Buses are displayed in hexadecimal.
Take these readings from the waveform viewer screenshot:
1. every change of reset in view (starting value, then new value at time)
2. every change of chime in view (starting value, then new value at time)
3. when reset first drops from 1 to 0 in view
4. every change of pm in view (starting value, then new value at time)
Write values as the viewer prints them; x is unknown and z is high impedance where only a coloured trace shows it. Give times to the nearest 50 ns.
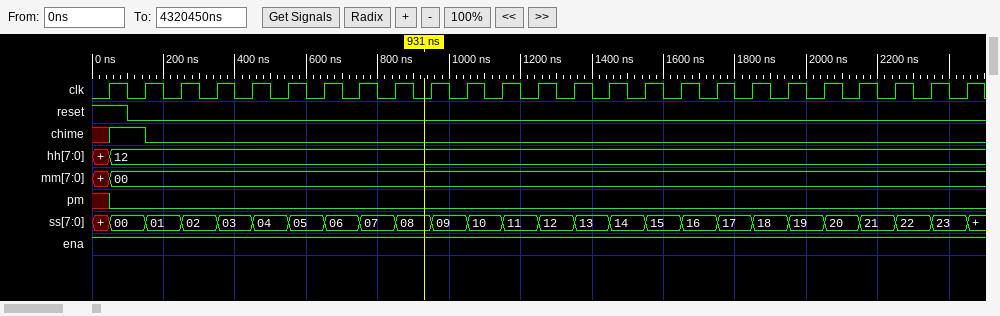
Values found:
1, 0 at 100 ns
x, 1 at 50 ns, 0 at 150 ns
100 ns
x, 0 at 50 ns
